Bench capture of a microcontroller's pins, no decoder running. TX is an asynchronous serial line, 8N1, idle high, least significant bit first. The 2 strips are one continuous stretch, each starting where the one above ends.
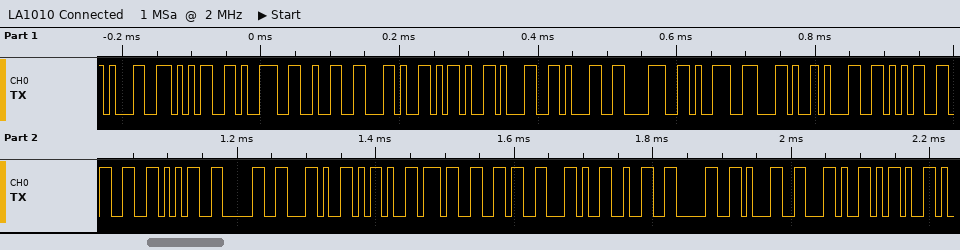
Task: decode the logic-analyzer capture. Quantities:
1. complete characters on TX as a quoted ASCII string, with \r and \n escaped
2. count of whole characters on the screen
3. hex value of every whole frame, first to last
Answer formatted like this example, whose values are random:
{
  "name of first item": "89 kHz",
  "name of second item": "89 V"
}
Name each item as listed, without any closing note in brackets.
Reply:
{
  "complete characters on TX as a quoted ASCII string, with \\r and \\n escaped": "\"1592,-1189,15350,-76,201,-\"",
  "count of whole characters on the screen": "26",
  "hex value of every whole frame, first to last": "0x31 0x35 0x39 0x32 0x2C 0x2D 0x31 0x31 0x38 0x39 0x2C 0x31 0x35 0x33 0x35 0x30 0x2C 0x2D 0x37 0x36 0x2C 0x32 0x30 0x31 0x2C 0x2D"
}
